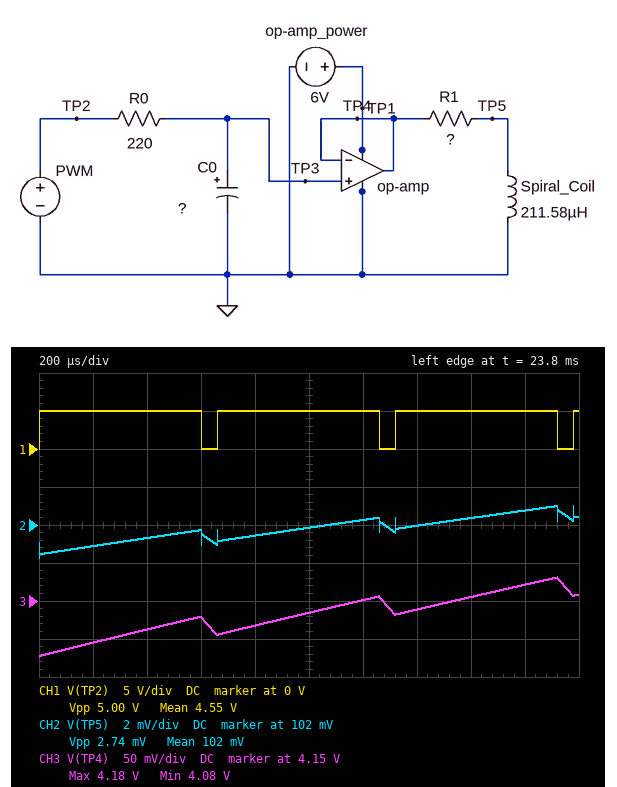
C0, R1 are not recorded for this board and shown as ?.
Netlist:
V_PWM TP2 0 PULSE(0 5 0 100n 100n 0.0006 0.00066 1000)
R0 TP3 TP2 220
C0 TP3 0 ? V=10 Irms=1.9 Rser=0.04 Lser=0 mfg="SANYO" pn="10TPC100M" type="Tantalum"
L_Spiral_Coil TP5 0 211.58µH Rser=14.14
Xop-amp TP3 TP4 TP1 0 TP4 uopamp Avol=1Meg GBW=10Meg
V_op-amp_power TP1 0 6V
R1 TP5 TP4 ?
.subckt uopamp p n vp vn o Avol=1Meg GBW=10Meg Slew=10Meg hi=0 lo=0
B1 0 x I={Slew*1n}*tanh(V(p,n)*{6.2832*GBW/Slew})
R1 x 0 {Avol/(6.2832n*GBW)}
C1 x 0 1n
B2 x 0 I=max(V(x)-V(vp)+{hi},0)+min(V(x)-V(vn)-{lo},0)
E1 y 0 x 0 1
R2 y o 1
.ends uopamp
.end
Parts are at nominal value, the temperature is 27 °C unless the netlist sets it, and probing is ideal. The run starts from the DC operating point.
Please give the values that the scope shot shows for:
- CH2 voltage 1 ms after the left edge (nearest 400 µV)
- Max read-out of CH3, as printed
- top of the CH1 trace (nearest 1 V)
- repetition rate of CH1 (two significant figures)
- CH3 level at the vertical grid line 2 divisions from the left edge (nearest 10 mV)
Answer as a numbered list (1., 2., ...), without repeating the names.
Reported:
1. 102.0 mV
2. 4.18 V
3. 5 V
4. 1.5 kHz
5. 4.11 V
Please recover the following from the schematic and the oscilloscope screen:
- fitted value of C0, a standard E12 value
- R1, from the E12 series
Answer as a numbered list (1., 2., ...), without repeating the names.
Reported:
1. 47 µF
2. 560 Ω
